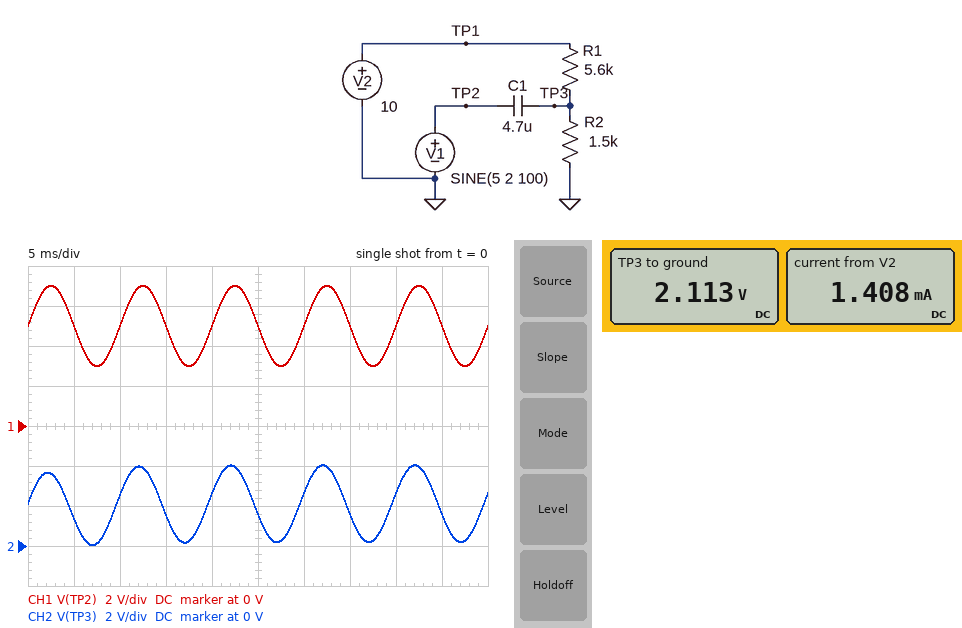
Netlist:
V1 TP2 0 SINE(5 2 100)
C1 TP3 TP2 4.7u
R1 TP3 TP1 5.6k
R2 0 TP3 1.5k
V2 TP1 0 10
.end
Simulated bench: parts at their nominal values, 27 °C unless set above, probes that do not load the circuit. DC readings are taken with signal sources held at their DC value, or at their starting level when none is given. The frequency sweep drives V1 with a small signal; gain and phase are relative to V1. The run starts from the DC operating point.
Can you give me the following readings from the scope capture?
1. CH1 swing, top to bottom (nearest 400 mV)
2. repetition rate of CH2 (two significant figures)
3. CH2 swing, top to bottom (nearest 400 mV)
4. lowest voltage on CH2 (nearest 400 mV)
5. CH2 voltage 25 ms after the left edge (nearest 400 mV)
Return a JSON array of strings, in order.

["4.0 V", "100 Hz", "4.0 V", "0 V", "1.6 V"]
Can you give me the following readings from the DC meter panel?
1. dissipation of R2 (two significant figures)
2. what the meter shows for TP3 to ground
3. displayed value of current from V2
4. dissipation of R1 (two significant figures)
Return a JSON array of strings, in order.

["3.0 mW", "2.113 V", "1.408 mA", "11 mW"]
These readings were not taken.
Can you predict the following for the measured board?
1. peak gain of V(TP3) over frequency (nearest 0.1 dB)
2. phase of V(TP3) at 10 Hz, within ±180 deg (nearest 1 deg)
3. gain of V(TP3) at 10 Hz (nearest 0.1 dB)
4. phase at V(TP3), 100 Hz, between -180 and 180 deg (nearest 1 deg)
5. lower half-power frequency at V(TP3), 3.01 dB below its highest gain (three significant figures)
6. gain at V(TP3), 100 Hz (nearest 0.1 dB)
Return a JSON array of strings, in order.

["0 dB", "71 deg", "-9.6 dB", "16 deg", "28.6 Hz", "-0.3 dB"]
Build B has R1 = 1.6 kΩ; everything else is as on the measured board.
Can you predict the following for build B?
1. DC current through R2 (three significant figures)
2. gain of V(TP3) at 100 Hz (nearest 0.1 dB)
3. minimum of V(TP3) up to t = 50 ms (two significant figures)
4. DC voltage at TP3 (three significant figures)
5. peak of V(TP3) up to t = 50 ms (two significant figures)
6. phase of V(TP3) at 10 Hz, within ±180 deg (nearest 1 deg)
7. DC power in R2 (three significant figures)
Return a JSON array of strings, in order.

["3.23 mA", "-0.8 dB", "2.9 V", "4.84 V", "6.7 V", "77 deg", "15.6 mW"]
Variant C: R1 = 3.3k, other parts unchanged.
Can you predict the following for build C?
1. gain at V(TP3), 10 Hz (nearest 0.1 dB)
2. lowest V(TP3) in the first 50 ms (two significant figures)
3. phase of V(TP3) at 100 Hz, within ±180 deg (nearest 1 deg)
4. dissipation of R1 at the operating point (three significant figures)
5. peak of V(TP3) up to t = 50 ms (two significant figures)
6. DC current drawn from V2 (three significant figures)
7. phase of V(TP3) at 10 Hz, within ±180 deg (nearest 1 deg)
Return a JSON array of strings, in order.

["-10.7 dB", "1.1 V", "18 deg", "14.3 mW", "5.0 V", "2.08 mA", "73 deg"]
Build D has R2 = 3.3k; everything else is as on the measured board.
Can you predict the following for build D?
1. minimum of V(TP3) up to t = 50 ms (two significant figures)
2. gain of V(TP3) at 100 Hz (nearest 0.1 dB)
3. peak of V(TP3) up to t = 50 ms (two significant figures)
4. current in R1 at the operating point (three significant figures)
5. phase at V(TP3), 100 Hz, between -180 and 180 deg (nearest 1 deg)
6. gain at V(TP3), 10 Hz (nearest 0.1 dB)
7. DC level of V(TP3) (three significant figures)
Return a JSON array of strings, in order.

["1.6 V", "-0.1 dB", "5.7 V", "1.12 mA", "9 deg", "-5.6 dB", "3.71 V"]
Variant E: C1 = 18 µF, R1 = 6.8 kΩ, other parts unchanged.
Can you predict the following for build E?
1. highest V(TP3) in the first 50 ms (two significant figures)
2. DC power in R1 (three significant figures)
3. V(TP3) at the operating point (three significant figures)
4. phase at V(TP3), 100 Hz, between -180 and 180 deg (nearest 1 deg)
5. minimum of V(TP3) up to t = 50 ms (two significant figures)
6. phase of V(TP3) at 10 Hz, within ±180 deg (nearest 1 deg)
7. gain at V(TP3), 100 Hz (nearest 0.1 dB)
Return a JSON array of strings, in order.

["3.8 V", "9.87 mW", "1.81 V", "4 deg", "-290 mV", "36 deg", "0 dB"]
